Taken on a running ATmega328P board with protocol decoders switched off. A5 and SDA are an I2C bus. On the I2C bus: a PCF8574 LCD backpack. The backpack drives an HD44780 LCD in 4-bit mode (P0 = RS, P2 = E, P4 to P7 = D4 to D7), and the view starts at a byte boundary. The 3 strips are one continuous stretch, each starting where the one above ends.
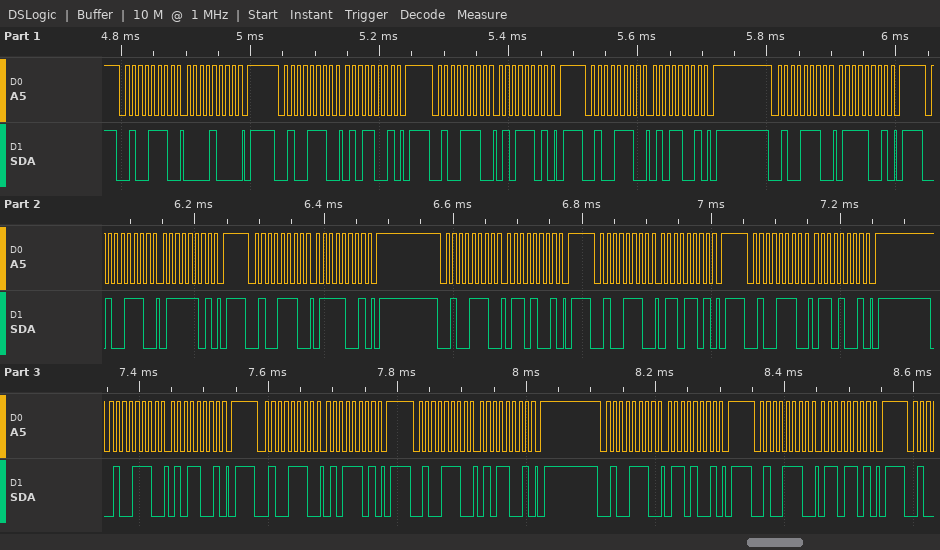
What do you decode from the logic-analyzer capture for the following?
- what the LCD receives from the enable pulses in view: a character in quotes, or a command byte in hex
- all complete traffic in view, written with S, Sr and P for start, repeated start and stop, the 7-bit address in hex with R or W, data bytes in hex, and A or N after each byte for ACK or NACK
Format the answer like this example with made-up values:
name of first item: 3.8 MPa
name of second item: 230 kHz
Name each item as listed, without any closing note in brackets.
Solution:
what the LCD receives from the enable pulses in view: a character in quotes, or a command byte in hex: 'W' 'e'
all complete traffic in view, written with S, Sr and P for start, repeated start and stop, the 7-bit address in hex with R or W, data bytes in hex, and A or N after each byte for ACK or NACK: S 27W A 08 A P S 27W A 59 A P S 27W A 5D A P S 27W A 59 A P S 27W A 79 A P S 27W A 7D A P S 27W A 79 A P S 27W A 69 A P S 27W A 6D A P S 27W A 69 A P S 27W A 59 A P S 27W A 5D A P S 27W A 59 A P S 27W A 69 A P S 27W A 6D A P
